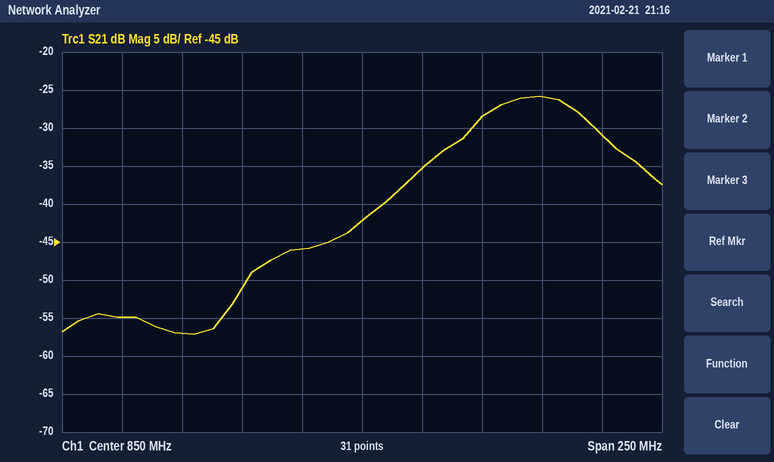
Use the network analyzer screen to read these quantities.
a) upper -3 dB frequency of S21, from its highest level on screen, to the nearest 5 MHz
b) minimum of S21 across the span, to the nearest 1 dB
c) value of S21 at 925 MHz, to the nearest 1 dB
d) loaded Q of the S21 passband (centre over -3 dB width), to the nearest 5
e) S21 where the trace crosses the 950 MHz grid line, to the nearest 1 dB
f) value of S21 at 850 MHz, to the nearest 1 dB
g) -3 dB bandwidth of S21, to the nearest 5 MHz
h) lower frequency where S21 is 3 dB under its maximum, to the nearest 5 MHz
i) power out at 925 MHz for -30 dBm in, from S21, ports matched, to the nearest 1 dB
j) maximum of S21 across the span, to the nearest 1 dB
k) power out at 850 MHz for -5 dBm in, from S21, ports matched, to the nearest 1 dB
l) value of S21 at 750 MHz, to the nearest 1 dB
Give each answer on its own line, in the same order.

945 MHz
-57 dB
-26 dB
20
-31 dB
-42 dB
45 MHz
900 MHz
-56 dBm
-26 dB
-47 dBm
-55 dB
